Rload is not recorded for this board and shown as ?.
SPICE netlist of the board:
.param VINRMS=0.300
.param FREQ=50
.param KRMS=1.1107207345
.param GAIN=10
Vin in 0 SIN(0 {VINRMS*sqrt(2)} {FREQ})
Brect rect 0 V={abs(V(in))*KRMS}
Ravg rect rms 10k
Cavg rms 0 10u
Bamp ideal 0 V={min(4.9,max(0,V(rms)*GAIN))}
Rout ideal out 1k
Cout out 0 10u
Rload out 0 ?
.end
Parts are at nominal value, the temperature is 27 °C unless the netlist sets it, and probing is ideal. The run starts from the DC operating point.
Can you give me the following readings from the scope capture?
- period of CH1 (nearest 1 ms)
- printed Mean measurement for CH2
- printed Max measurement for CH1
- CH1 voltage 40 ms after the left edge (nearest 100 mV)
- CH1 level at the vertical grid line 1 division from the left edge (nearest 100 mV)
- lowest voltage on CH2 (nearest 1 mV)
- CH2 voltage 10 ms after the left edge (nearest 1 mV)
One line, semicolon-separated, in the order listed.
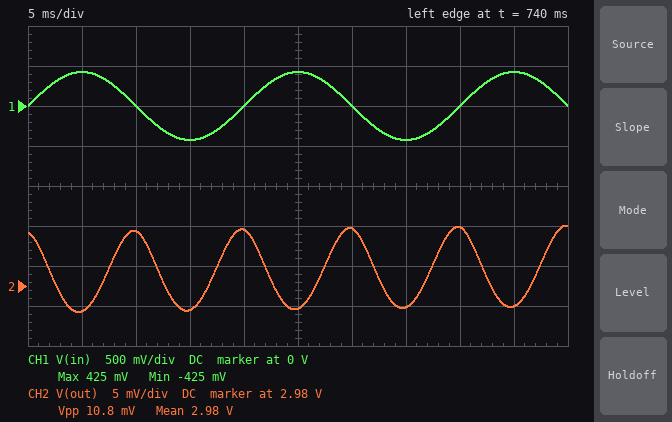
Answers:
20 ms; 2.98 V; 425 mV; 0 V; 400 mV; 2.977 V; 2.987 V
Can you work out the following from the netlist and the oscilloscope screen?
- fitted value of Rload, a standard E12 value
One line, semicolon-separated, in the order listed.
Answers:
180 kΩ
